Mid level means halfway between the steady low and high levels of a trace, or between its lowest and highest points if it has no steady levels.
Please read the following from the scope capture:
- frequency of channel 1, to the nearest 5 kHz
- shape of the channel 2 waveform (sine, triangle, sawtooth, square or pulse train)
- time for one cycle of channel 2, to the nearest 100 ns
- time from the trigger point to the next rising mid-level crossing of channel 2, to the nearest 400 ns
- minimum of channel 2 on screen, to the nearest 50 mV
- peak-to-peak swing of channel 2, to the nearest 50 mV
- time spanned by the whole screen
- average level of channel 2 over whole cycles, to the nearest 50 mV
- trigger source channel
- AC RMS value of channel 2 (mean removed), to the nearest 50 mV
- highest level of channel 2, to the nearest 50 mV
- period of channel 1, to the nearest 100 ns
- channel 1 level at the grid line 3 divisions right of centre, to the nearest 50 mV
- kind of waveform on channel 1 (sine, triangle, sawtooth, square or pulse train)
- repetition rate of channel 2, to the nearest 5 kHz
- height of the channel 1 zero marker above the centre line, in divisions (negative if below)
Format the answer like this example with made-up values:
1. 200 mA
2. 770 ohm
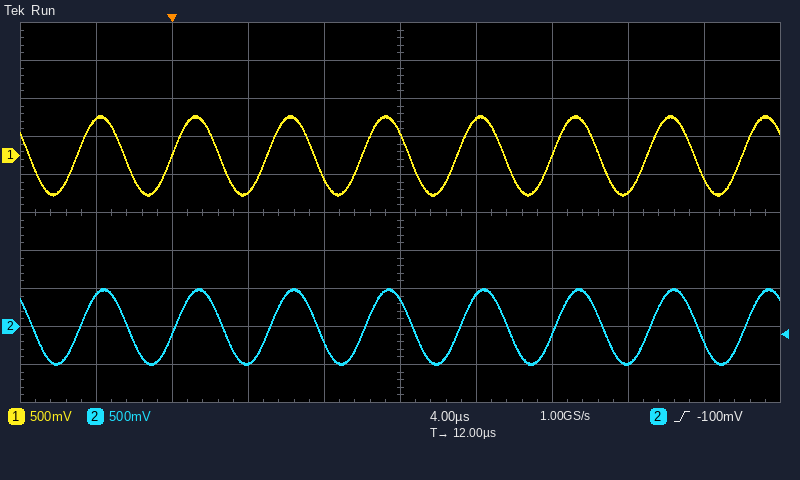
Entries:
1. 200 kHz
2. sine
3. 5.0 µs
4. 5.2 µs
5. -500 mV
6. 1.00 V
7. 40 µs
8. 0 mV
9. channel 2
10. 350 mV
11. 500 mV
12. 5.0 µs
13. -450 mV
14. sine
15. 200 kHz
16. +1.5 div
